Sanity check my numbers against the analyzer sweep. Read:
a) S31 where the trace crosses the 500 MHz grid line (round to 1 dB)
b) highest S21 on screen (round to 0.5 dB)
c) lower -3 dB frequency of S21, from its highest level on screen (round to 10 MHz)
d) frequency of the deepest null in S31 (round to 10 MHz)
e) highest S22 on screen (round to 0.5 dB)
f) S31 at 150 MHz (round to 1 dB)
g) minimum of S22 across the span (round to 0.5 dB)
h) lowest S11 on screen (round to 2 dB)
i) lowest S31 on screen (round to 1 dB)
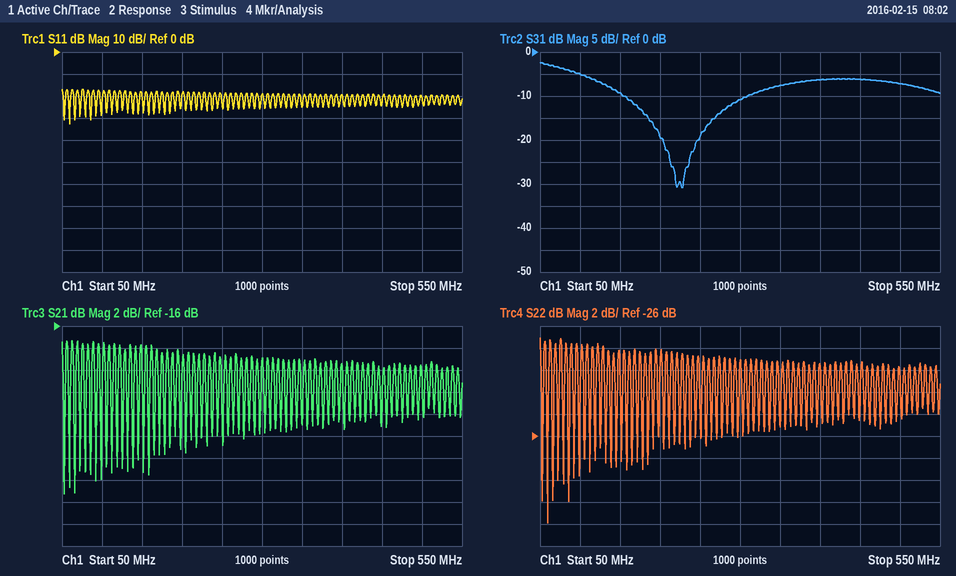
-7 dB
-17.5 dB
60 MHz
230 MHz
-17.0 dB
-9 dB
-34.0 dB
-32 dB
-31 dB
